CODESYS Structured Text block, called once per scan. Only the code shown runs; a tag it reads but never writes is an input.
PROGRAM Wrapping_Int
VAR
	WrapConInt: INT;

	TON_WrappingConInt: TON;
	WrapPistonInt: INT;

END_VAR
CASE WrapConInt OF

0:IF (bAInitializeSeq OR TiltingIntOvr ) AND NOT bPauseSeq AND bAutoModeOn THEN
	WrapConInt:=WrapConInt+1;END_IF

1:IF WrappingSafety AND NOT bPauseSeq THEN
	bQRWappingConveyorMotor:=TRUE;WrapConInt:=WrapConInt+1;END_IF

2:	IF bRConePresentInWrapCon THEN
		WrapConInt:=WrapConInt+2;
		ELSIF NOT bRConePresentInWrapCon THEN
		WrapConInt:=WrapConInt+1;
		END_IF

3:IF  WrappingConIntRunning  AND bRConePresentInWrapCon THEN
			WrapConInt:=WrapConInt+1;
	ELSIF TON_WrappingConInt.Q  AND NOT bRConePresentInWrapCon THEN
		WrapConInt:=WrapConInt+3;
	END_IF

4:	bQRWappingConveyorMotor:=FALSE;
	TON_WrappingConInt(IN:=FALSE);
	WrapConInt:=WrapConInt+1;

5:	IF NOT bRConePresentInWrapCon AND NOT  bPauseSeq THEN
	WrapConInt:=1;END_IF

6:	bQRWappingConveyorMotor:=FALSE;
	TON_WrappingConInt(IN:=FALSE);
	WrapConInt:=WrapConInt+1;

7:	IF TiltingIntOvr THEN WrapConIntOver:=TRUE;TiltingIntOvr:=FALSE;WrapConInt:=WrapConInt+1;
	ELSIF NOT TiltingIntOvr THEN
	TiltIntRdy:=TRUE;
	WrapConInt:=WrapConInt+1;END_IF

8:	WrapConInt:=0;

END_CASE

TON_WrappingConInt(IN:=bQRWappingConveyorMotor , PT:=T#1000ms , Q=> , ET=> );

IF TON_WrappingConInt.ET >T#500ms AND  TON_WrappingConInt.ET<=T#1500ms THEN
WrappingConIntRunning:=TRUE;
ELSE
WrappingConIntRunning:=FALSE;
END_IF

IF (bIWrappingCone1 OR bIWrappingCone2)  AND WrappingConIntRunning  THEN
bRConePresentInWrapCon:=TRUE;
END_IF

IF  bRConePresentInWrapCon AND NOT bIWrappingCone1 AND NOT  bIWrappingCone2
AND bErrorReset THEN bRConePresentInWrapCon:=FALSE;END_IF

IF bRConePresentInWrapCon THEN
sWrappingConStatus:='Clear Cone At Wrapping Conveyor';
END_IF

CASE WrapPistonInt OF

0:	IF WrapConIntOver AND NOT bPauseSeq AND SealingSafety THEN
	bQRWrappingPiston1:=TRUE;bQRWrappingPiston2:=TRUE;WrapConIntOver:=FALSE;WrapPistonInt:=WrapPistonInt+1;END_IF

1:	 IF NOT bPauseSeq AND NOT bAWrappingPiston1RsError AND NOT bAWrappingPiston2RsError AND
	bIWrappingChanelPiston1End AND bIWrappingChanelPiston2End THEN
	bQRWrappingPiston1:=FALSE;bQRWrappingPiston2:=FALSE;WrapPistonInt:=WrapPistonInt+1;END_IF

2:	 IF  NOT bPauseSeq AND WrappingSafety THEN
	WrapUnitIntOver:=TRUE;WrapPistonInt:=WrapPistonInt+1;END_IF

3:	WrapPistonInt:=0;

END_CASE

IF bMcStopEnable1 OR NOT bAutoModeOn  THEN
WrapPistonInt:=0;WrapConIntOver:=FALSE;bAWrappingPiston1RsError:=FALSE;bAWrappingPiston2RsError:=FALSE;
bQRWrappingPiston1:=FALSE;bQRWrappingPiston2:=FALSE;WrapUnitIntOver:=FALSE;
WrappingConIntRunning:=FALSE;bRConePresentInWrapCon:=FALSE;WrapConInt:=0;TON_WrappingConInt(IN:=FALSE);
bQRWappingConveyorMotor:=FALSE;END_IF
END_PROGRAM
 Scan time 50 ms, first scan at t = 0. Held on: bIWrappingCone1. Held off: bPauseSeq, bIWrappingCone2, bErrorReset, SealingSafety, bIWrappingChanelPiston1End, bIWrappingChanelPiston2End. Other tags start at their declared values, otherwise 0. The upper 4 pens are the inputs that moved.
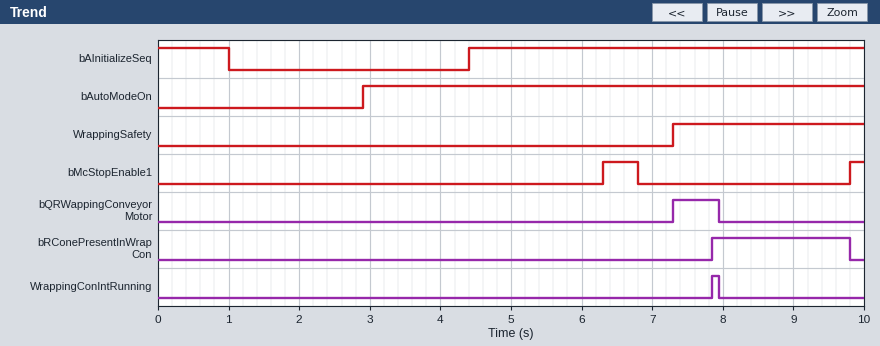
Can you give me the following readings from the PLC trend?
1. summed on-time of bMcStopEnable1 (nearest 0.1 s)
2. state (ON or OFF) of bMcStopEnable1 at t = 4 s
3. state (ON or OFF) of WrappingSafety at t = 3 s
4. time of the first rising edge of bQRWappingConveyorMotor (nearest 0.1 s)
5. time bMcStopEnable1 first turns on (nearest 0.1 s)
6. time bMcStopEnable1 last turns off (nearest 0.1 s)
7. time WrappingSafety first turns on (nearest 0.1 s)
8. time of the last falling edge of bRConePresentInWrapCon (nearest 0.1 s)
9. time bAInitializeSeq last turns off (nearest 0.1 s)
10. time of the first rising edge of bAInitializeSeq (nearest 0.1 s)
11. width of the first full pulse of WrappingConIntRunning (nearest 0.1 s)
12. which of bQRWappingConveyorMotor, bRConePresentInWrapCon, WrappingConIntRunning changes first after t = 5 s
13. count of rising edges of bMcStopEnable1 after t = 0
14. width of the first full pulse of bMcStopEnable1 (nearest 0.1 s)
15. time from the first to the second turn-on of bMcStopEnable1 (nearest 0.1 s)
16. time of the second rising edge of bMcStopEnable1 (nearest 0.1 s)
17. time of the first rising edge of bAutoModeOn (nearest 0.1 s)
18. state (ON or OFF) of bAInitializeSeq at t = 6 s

0.7 s
OFF
OFF
7.3 s
6.3 s
6.8 s
7.3 s
9.8 s
1.0 s
4.4 s
0.1 s
bQRWappingConveyorMotor
2
0.5 s
3.5 s
9.8 s
2.9 s
ON
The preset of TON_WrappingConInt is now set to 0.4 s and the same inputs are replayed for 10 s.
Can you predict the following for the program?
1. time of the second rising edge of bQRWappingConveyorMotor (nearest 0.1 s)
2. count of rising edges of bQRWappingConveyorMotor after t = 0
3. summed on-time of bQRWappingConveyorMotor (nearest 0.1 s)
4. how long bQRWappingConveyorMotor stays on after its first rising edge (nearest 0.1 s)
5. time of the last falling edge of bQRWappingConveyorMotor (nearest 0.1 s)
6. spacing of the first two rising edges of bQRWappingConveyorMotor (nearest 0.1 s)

8.0 s
4
1.9 s
0.5 s
9.8 s
0.7 s
